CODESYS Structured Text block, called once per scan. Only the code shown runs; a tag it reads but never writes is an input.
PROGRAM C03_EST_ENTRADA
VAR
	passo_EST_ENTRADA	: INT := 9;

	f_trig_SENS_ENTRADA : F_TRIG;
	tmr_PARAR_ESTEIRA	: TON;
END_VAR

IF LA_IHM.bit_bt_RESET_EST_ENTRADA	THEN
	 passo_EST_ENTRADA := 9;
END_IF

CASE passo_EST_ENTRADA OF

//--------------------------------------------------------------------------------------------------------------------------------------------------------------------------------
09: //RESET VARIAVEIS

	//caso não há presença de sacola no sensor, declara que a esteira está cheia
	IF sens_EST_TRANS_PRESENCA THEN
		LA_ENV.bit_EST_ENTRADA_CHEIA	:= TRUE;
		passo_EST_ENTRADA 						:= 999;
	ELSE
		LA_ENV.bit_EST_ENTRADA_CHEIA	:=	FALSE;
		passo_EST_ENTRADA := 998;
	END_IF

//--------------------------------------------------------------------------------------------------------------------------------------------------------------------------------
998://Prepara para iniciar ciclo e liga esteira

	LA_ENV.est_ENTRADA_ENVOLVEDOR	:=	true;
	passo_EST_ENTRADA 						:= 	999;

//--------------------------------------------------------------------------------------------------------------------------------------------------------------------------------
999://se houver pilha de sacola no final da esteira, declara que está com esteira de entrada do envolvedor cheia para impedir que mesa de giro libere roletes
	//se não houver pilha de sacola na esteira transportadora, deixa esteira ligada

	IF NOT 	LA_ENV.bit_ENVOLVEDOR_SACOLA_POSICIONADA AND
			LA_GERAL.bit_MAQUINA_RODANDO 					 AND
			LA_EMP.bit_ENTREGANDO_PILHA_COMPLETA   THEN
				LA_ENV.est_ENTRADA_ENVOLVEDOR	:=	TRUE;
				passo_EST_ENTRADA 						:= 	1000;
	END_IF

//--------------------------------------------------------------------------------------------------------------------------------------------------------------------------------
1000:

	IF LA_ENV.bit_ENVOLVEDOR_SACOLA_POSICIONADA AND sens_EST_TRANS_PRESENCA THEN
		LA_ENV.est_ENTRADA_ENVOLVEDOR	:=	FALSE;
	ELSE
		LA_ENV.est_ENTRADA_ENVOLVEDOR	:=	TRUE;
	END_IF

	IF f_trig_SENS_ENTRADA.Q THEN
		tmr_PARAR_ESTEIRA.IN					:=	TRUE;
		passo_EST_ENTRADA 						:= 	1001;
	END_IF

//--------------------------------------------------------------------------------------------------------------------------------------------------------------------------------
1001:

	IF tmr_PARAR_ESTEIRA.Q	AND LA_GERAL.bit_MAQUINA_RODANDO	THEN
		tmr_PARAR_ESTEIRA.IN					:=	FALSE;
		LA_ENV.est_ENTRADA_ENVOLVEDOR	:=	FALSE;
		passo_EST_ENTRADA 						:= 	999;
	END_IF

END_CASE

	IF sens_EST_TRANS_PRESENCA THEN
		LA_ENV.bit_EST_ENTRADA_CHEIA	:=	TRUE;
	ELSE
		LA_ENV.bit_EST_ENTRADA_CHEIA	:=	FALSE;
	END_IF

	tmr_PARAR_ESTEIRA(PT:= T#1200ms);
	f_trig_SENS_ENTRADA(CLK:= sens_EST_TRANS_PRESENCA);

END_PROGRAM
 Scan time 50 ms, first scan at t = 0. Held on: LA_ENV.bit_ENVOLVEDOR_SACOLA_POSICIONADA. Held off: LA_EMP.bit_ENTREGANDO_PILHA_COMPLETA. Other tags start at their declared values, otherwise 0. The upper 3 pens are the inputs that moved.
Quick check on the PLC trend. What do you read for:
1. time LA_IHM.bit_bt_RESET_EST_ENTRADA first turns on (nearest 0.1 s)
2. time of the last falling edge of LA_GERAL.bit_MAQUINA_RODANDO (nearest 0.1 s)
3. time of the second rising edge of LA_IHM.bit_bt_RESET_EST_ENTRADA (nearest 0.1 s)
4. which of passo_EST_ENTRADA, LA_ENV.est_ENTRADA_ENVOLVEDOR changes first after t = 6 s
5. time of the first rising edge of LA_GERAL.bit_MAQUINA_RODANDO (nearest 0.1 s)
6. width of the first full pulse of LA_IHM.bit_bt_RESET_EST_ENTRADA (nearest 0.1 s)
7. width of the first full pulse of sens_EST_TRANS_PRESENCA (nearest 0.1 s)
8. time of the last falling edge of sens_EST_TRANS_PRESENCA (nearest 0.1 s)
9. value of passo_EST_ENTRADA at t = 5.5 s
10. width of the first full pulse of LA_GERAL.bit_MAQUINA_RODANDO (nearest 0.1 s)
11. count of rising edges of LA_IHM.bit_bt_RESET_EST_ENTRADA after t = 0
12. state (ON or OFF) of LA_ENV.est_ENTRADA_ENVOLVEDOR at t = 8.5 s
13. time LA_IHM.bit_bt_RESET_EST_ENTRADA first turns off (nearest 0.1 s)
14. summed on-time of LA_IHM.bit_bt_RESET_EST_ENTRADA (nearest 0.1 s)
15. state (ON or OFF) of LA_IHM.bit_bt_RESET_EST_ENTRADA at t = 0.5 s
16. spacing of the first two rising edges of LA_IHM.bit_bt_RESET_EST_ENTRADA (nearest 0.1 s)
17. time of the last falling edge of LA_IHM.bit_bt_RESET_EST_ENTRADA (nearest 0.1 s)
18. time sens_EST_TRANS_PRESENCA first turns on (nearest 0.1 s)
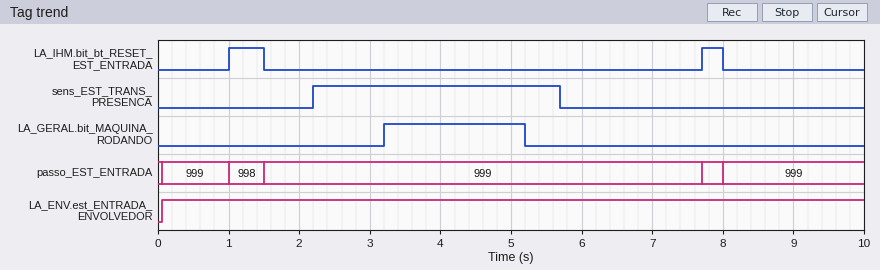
1.0 s
5.2 s
7.7 s
passo_EST_ENTRADA
3.2 s
0.5 s
3.5 s
5.7 s
999
2.0 s
2
ON
1.5 s
0.8 s
OFF
6.7 s
8.0 s
2.2 s
